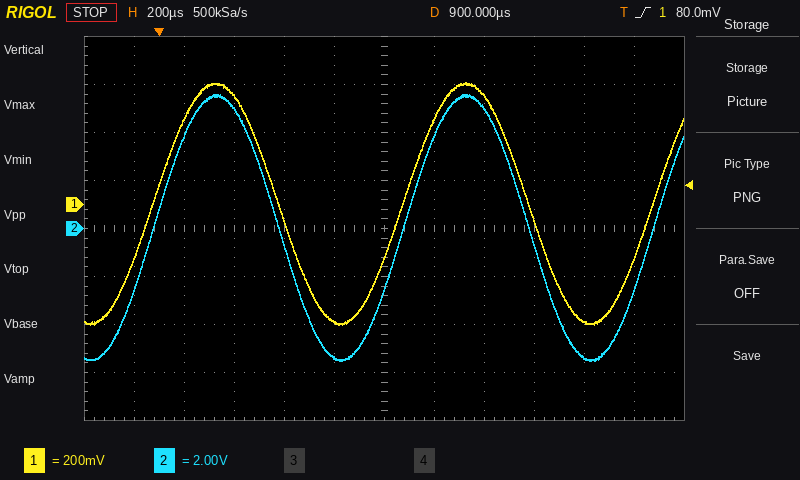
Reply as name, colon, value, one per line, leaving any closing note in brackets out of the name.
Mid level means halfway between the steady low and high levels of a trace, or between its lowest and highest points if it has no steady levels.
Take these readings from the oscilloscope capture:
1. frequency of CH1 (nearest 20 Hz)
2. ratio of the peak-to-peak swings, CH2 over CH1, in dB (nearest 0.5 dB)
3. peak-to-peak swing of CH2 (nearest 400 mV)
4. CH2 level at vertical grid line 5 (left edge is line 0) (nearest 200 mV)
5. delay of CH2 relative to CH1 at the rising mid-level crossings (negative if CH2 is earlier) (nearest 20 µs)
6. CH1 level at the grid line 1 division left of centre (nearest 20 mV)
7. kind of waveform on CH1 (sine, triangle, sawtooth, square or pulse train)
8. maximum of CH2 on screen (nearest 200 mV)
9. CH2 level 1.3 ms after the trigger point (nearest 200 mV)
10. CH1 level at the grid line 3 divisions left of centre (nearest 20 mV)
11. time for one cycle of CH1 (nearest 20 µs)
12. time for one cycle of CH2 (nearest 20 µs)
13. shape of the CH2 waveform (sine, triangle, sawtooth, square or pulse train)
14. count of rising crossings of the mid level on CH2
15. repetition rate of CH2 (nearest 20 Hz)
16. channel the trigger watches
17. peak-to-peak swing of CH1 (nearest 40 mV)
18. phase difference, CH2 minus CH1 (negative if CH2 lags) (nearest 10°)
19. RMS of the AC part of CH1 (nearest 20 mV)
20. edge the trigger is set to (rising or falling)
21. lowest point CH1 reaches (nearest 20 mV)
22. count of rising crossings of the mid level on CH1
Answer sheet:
frequency of CH1: 1.00 kHz
ratio of the peak-to-peak swings, CH2 over CH1, in dB: 21.0 dB
peak-to-peak swing of CH2: 11.2 V
CH2 level at vertical grid line 5 (left edge is line 0): -5.4 V
delay of CH2 relative to CH1 at the rising mid-level crossings (negative if CH2 is earlier): 0 µs
CH1 level at the grid line 1 division left of centre: -480 mV
kind of waveform on CH1: sine
maximum of CH2 on screen: 5.6 V
CH2 level 1.3 ms after the trigger point: 5.0 V
CH1 level at the grid line 3 divisions left of centre: 460 mV
time for one cycle of CH1: 1.00 ms
time for one cycle of CH2: 1.00 ms
shape of the CH2 waveform: sine
count of rising crossings of the mid level on CH2: 3
repetition rate of CH2: 1.00 kHz
channel the trigger watches: CH1
peak-to-peak swing of CH1: 1.00 V
phase difference, CH2 minus CH1 (negative if CH2 lags): 0°
RMS of the AC part of CH1: 360 mV
edge the trigger is set to: rising
lowest point CH1 reaches: -500 mV
count of rising crossings of the mid level on CH1: 3
